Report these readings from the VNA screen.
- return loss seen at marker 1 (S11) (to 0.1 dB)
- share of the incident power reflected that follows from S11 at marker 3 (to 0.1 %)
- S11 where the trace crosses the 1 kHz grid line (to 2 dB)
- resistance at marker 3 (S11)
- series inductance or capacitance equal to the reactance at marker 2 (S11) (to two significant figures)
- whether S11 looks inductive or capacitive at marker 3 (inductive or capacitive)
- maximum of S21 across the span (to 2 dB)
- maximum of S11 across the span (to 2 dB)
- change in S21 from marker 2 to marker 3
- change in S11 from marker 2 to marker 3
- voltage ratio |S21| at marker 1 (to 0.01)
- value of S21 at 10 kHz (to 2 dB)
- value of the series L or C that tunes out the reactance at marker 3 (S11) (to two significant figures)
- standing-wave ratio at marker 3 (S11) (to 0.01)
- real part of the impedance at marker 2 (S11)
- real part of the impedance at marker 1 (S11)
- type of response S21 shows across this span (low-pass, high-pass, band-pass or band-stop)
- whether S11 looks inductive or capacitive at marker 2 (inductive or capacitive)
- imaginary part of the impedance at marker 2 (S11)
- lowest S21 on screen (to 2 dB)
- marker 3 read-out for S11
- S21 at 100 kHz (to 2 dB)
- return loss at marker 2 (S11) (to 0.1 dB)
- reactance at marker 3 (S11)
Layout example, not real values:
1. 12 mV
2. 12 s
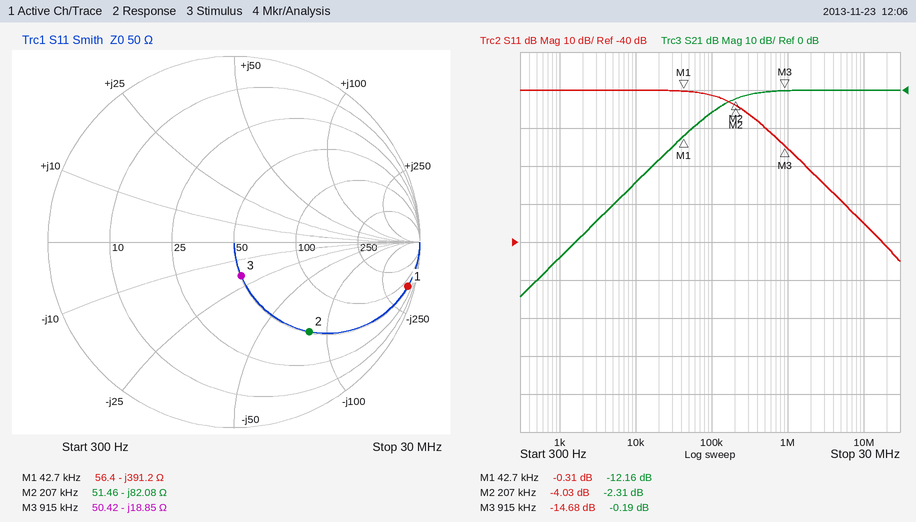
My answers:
1. 0.3 dB
2. 3.4 %
3. 0 dB
4. 50.42 Ω
5. 9.4 nF
6. capacitive
7. 0 dB
8. 0 dB
9. 2.12 dB
10. -10.65 dB
11. 0.25
12. -24 dB
13. 3.3 µH
14. 1.45
15. 51.46 Ω
16. 56.4 Ω
17. high-pass
18. capacitive
19. -82.08 Ω
20. -54 dB
21. -14.68 dB
22. -6 dB
23. 4.0 dB
24. -18.85 Ω
